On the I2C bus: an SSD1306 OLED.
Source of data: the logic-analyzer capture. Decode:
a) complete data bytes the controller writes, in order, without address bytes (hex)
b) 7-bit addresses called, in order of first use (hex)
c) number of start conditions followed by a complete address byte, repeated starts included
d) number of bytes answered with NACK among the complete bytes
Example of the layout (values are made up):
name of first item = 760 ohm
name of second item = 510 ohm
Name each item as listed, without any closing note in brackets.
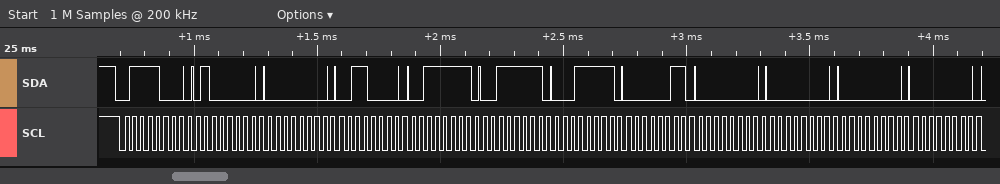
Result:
complete data bytes the controller writes, in order, without address bytes = 40 00 30 3F 3F 1F 03 00 00 00 00
7-bit addresses called, in order of first use = 0x3C
number of start conditions followed by a complete address byte, repeated starts included = 1
number of bytes answered with NACK among the complete bytes = 0
